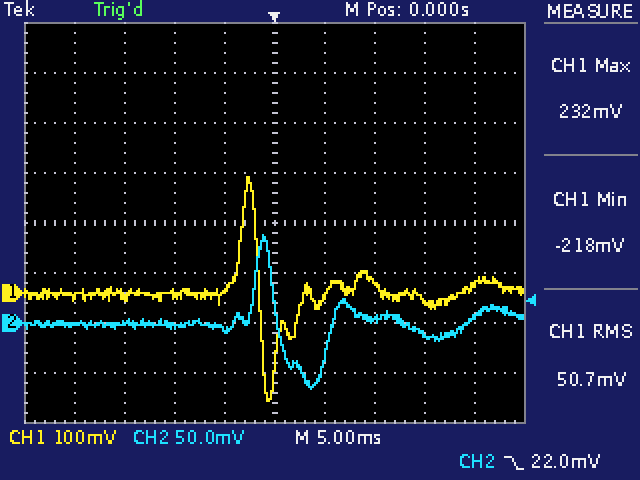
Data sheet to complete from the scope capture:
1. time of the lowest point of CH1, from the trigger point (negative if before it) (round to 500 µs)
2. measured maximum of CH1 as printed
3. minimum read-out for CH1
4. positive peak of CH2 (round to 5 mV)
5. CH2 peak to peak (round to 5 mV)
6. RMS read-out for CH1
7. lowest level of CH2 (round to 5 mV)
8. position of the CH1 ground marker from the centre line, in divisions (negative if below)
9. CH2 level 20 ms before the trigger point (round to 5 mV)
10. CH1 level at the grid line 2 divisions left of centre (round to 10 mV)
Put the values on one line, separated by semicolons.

-500 µs; 232 mV; -218 mV; 90 mV; 155 mV; 50.7 mV; -65 mV; -1.4 div; 0 mV; 0 mV
